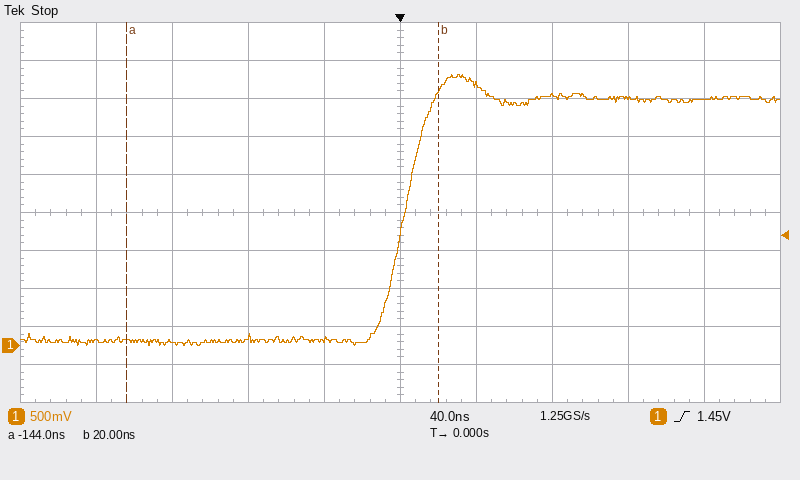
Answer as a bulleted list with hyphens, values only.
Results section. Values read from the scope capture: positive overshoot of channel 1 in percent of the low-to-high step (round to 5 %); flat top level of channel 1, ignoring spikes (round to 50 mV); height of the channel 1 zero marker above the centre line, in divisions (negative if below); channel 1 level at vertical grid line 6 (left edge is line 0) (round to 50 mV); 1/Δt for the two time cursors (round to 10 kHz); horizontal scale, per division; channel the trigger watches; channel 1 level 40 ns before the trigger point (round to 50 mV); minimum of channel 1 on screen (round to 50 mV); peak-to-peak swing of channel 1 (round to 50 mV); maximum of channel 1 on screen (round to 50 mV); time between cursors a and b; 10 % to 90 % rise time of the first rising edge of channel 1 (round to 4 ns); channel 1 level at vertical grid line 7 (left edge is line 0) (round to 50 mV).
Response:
- 10 %
- 3.25 V
- -3.5 div
- 3.45 V
- 6.10 MHz
- 40 ns
- channel 1
- 100 mV
- 0 mV
- 3.55 V
- 3.55 V
- 164 ns
- 24 ns
- 3.30 V
